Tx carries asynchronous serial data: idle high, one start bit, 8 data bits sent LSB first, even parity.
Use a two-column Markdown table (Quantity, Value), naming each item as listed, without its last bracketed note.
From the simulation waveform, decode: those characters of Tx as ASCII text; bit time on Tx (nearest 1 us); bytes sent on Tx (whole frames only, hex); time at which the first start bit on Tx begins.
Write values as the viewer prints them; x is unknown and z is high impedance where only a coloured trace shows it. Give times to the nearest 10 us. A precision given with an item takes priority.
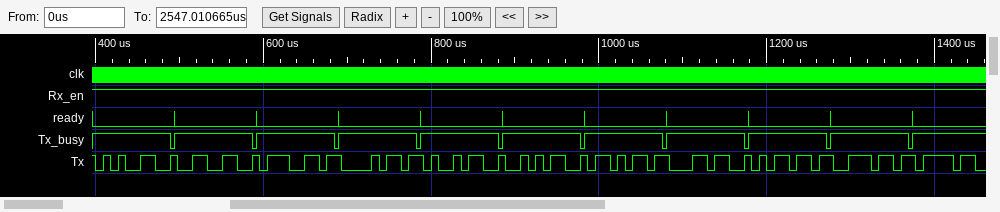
| Quantity | Value |
|---|---|
| those characters of Tx as ASCII text | "efghijklmn" |
| bit time on Tx | 9 us |
| bytes sent on Tx | 65, 66, 67, 68, 69, 6A, 6B, 6C, 6D, 6E |
| time at which the first start bit on Tx begins | 400 us |
